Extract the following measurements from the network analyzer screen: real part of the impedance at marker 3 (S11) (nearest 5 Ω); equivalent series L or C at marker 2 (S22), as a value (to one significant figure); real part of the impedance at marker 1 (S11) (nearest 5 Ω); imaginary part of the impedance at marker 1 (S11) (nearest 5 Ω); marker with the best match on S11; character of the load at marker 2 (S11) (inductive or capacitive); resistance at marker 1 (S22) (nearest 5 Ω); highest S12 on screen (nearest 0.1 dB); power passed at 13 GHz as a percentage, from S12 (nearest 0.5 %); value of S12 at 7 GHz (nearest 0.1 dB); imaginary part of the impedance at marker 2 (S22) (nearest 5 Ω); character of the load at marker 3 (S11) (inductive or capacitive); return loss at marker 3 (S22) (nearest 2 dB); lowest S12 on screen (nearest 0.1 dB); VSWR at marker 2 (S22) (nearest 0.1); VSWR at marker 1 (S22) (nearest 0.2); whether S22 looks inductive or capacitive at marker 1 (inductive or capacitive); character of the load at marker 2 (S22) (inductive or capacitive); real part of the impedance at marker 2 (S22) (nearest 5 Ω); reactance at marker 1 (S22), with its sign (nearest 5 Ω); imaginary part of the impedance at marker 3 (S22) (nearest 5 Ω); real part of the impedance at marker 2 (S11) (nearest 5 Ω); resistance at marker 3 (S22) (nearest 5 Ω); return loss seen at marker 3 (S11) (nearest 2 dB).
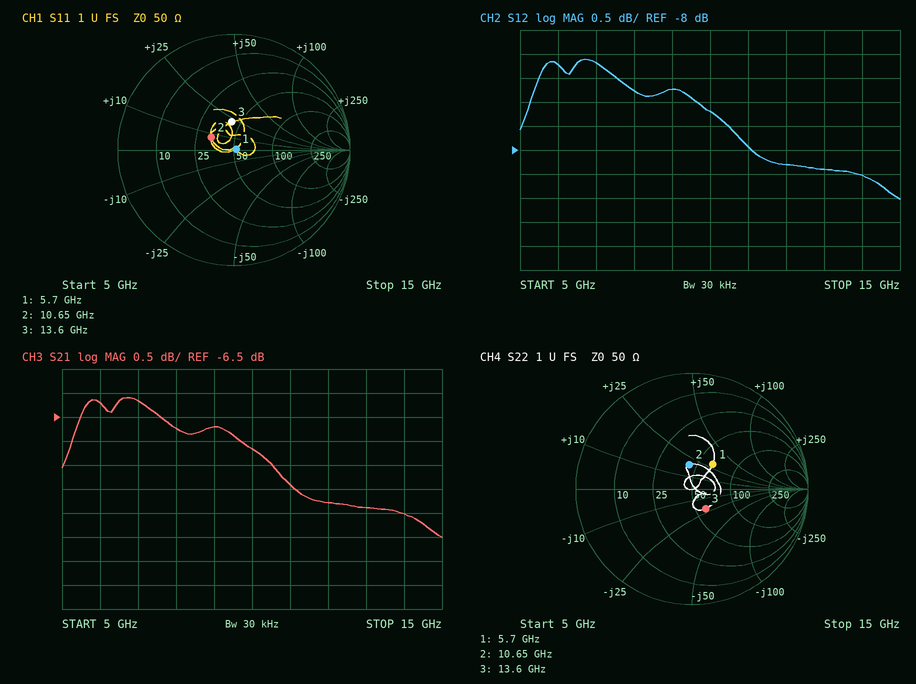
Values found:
45 Ω
300 pH
50 Ω
0 Ω
marker 1
inductive
65 Ω
-6.1 dB
14.5 %
-6.2 dB
+20 Ω
inductive
14 dB
-9.0 dB
1.5
1.8
inductive
inductive
45 Ω
+30 Ω
-20 Ω
35 Ω
60 Ω
12 dB
